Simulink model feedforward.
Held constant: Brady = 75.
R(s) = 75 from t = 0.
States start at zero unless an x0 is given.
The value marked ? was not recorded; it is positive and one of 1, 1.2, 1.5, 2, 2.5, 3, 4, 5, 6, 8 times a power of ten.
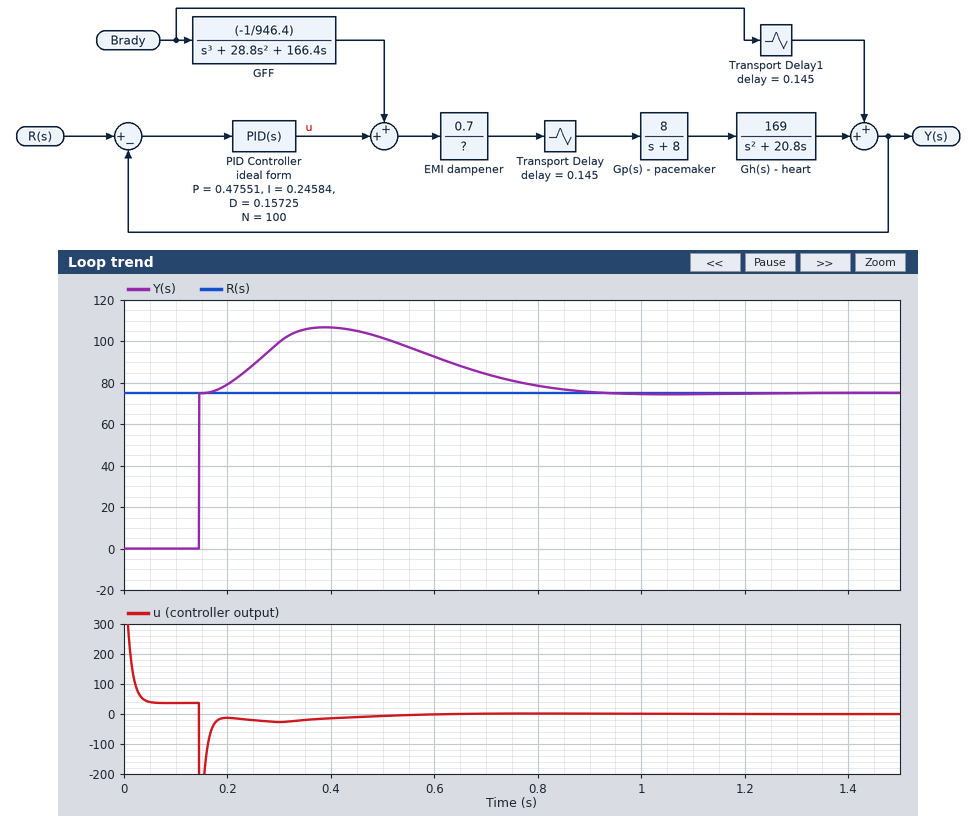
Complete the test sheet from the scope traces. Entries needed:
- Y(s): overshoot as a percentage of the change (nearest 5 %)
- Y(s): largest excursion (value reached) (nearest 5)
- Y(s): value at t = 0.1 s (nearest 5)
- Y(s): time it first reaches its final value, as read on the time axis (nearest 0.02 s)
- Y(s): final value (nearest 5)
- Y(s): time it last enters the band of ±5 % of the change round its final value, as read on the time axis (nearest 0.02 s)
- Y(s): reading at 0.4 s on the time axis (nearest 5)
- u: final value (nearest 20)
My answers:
45 %
105
0
0.14 s
75
0.80 s
105
0
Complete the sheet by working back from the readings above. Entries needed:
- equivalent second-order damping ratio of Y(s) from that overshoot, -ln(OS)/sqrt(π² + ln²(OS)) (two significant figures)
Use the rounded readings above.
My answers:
0.25
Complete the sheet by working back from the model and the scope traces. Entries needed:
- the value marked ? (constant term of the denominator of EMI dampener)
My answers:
1
